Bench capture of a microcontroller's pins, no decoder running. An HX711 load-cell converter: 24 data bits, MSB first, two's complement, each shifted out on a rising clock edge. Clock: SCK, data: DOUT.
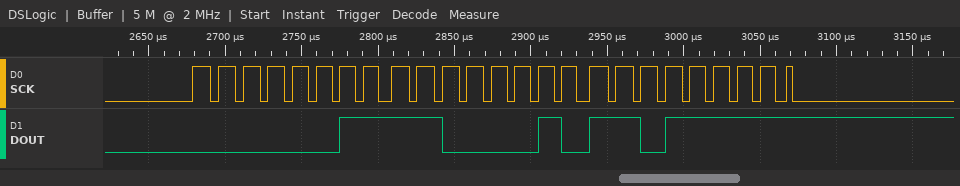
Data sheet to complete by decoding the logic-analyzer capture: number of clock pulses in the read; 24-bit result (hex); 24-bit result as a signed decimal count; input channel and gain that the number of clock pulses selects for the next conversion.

25
0x03C2DF
246495
channel A, gain 128
